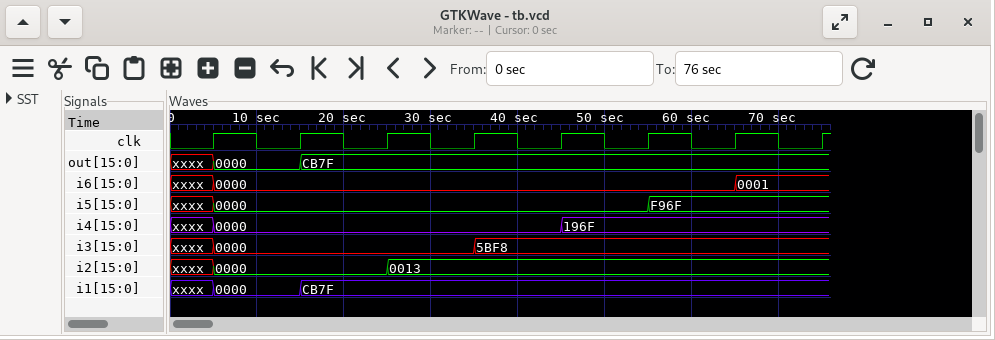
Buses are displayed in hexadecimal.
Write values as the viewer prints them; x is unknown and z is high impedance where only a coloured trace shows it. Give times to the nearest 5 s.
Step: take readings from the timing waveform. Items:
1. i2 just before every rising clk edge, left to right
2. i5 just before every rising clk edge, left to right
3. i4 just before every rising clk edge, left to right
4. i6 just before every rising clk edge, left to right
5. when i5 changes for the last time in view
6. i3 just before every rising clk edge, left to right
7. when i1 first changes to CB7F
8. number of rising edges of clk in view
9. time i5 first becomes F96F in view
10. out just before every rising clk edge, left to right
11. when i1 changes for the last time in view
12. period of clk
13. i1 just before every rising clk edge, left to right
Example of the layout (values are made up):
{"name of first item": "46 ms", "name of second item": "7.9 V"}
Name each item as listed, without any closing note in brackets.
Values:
{"i2 just before every rising clk edge, left to right": "xxxx, 0000, 0000, 0013, 0013, 0013, 0013, 0013", "i5 just before every rising clk edge, left to right": "xxxx, 0000, 0000, 0000, 0000, 0000, F96F, F96F", "i4 just before every rising clk edge, left to right": "xxxx, 0000, 0000, 0000, 0000, 196F, 196F, 196F", "i6 just before every rising clk edge, left to right": "xxxx, 0000, 0000, 0000, 0000, 0000, 0000, 0001", "when i5 changes for the last time in view": "55 s", "i3 just before every rising clk edge, left to right": "xxxx, 0000, 0000, 0000, 5BF8, 5BF8, 5BF8, 5BF8", "when i1 first changes to CB7F": "15 s", "number of rising edges of clk in view": "8", "time i5 first becomes F96F in view": "55 s", "out just before every rising clk edge, left to right": "xxxx, 0000, CB7F, CB7F, CB7F, CB7F, CB7F, CB7F", "when i1 changes for the last time in view": "15 s", "period of clk": "10 s", "i1 just before every rising clk edge, left to right": "xxxx, 0000, CB7F, CB7F, CB7F, CB7F, CB7F, CB7F"}
